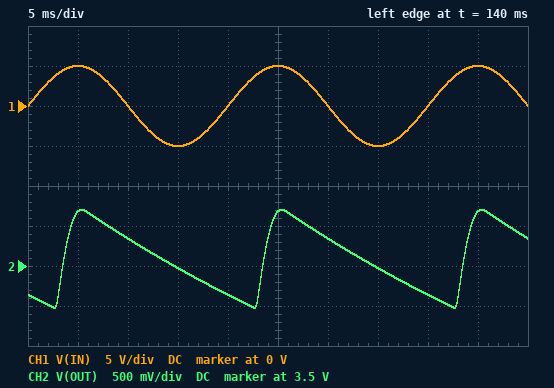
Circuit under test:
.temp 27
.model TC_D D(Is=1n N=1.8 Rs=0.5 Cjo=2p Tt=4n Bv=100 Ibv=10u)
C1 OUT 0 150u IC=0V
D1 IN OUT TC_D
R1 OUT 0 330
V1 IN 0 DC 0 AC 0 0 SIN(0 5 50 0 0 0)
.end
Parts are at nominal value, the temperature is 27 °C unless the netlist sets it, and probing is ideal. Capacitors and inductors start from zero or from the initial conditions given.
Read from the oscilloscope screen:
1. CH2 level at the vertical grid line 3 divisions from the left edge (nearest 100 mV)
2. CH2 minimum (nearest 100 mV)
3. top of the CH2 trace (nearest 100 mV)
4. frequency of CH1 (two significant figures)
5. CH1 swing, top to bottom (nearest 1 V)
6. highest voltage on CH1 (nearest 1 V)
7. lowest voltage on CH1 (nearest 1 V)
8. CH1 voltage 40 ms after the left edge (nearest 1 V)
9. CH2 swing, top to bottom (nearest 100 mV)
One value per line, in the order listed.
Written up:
3.5 V
3.0 V
4.2 V
50 Hz
10 V
5 V
-5 V
0 V
1.2 V
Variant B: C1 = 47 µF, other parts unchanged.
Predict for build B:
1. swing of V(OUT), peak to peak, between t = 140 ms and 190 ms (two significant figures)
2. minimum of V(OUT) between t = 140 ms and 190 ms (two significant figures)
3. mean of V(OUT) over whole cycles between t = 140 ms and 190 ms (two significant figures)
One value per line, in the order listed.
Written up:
2.7 V
1.5 V
2.8 V
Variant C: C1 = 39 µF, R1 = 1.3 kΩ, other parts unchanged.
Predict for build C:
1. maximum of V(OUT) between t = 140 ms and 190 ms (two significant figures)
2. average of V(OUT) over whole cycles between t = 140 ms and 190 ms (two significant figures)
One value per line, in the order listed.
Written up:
4.3 V
3.7 V
